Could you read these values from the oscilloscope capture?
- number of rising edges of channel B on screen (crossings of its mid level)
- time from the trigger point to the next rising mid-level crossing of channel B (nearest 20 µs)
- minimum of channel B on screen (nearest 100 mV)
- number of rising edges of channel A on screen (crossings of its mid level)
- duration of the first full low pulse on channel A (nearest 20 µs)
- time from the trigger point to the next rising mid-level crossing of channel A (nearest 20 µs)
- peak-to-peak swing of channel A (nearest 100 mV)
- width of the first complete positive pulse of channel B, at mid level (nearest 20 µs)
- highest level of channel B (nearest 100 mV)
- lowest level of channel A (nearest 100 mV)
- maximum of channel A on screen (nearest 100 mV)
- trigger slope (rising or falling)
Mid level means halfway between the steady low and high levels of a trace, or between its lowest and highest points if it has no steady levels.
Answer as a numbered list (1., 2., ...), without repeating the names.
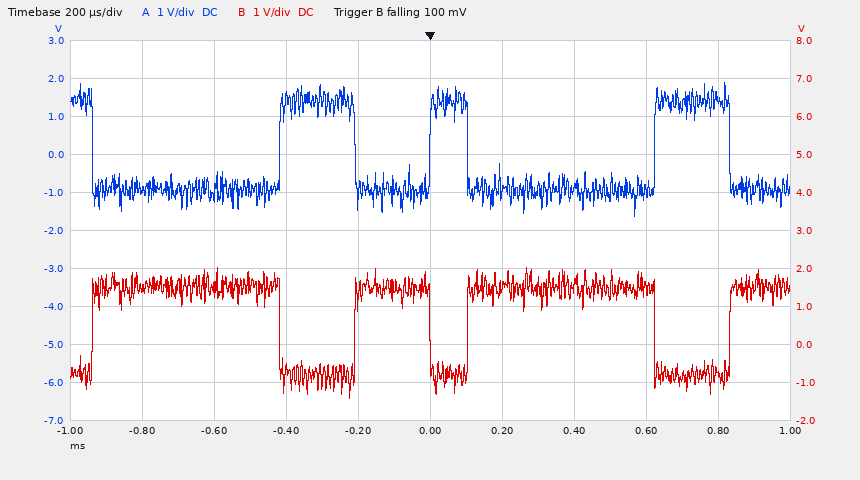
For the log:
1. 4
2. 100 µs
3. -1.4 V
4. 3
5. 520 µs
6. 620 µs
7. 3.5 V
8. 520 µs
9. 2.0 V
10. -1.6 V
11. 1.9 V
12. falling
